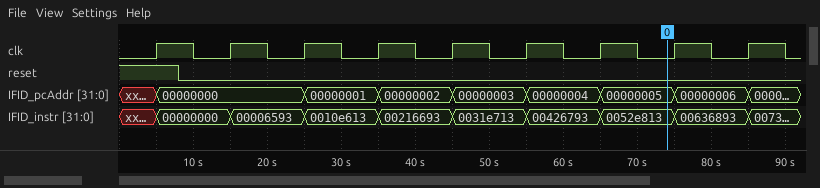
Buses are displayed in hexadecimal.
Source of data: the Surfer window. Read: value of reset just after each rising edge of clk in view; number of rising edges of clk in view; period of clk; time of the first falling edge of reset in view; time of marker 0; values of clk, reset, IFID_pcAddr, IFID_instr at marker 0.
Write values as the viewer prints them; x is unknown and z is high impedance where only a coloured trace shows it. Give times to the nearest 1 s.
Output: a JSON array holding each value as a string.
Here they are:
["1 0 0 0 0 0 0 0 0", "9", "10 s", "8 s", "74 s", "clk=0, reset=0, IFID_pcAddr=00000005, IFID_instr=0052e813"]
